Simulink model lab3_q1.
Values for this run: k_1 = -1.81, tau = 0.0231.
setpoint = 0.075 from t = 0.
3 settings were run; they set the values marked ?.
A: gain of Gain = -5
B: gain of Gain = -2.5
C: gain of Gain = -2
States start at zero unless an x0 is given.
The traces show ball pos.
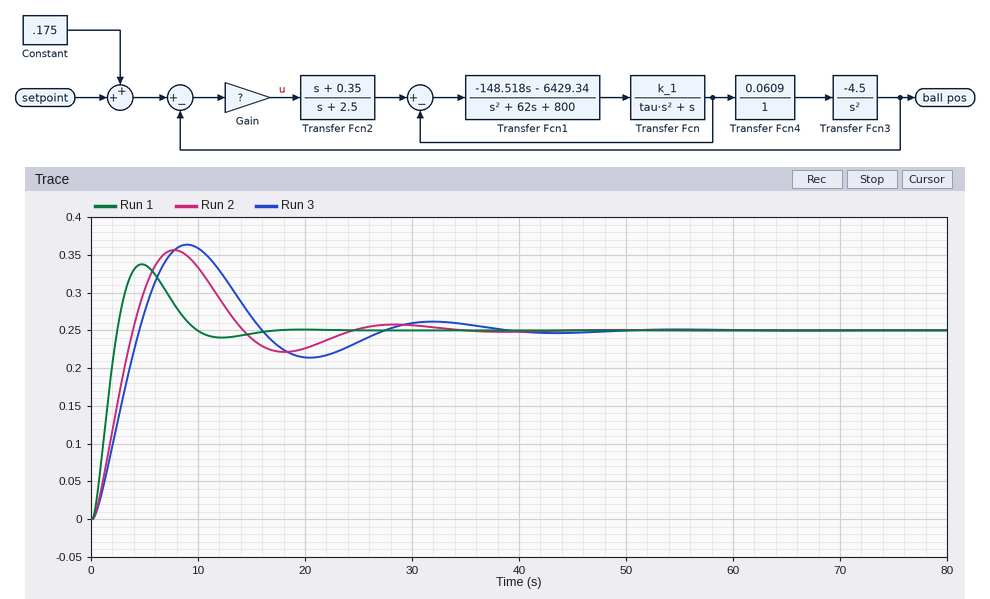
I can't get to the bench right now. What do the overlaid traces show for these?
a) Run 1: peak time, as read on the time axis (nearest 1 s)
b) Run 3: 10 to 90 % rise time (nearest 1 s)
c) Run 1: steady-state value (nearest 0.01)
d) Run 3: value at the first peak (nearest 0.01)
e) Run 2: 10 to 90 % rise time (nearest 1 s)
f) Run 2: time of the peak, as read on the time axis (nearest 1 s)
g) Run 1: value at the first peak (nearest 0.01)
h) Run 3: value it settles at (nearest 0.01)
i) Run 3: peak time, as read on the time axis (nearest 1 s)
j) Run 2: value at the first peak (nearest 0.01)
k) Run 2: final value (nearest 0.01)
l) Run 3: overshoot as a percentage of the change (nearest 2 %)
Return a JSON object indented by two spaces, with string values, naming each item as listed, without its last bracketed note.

{
  "Run 1: peak time, as read on the time axis": "5 s",
  "Run 3: 10 to 90 % rise time": "3 s",
  "Run 1: steady-state value": "0.25",
  "Run 3: value at the first peak": "0.36",
  "Run 2: 10 to 90 % rise time": "3 s",
  "Run 2: time of the peak, as read on the time axis": "8 s",
  "Run 1: value at the first peak": "0.34",
  "Run 3: value it settles at": "0.25",
  "Run 3: peak time, as read on the time axis": "9 s",
  "Run 2: value at the first peak": "0.36",
  "Run 2: final value": "0.25",
  "Run 3: overshoot as a percentage of the change": "46 %"
}
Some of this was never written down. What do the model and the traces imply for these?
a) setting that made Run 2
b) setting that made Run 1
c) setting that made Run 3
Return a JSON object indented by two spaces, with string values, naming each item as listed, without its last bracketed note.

{
  "setting that made Run 2": "B",
  "setting that made Run 1": "A",
  "setting that made Run 3": "C"
}
